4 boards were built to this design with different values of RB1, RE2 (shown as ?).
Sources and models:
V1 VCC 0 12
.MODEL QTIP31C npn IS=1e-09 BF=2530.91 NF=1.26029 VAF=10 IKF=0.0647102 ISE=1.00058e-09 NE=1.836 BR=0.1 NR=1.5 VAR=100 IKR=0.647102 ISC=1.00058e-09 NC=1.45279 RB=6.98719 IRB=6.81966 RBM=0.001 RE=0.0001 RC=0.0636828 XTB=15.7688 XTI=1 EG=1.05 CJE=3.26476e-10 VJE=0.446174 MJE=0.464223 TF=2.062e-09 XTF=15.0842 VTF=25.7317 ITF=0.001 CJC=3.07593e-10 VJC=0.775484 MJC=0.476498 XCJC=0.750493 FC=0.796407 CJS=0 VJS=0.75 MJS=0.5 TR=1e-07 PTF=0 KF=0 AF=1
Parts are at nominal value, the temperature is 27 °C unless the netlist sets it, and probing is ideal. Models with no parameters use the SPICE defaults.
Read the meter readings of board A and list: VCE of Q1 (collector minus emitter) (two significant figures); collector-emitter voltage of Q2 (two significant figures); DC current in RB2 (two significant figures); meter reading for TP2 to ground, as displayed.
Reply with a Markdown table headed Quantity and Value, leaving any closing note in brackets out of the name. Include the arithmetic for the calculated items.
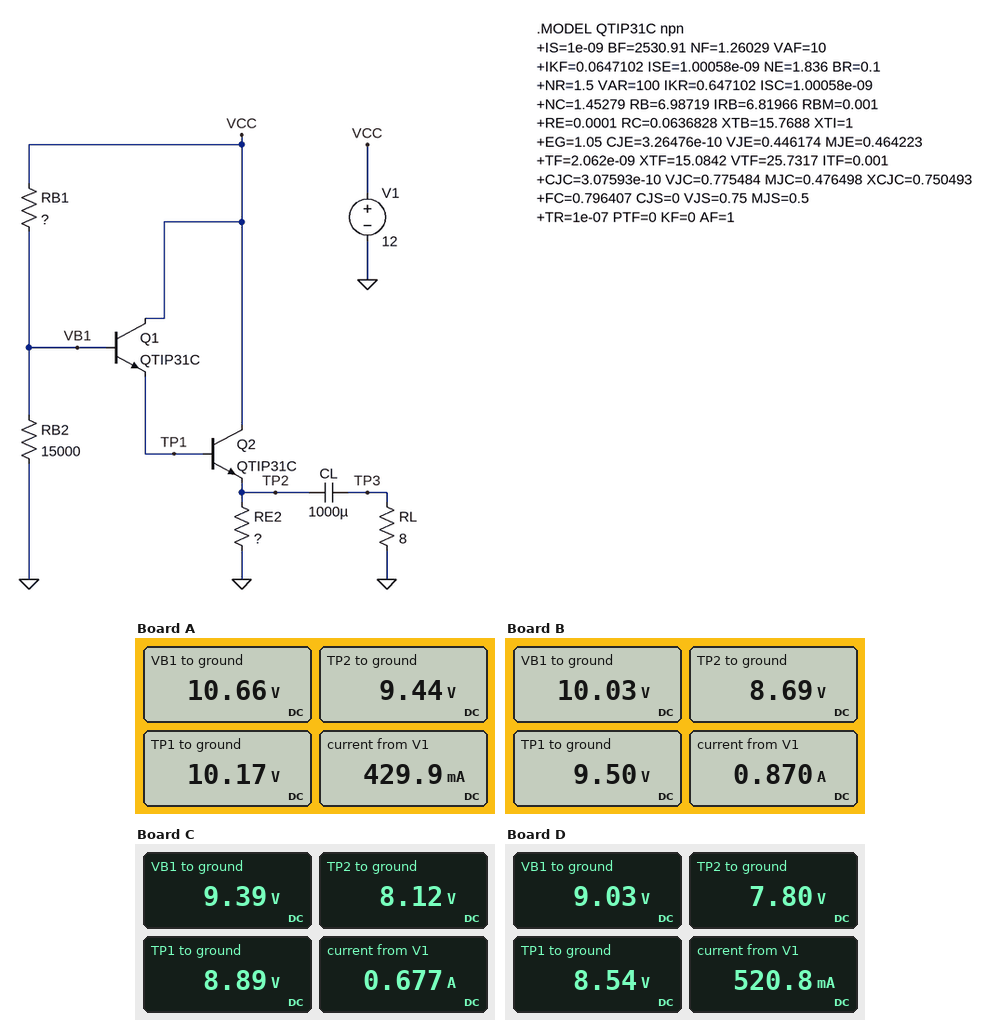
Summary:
| Quantity | Value |
|---|---|
| VCE of Q1 (collector minus emitter) | 12 V - 10.17 V = 1.8 V |
| collector-emitter voltage of Q2 | 12 V - 9.44 V = 2.6 V |
| DC current in RB2 | (10.66 V) / 15 kΩ = 710 µA |
| meter reading for TP2 to ground, as displayed | 9.44 V |
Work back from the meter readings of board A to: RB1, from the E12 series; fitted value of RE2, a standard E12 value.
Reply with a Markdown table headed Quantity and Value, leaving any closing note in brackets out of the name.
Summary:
| Quantity | Value |
|---|---|
| RB1, from the E12 series | 1.8 kΩ |
| fitted value of RE2, a standard E12 value | 22 Ω |
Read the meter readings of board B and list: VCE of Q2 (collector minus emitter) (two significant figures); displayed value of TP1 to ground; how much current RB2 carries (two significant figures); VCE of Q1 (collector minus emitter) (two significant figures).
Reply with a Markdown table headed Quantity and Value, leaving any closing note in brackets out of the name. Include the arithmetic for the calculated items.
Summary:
| Quantity | Value |
|---|---|
| VCE of Q2 (collector minus emitter) | 12 V - 8.69 V = 3.3 V |
| displayed value of TP1 to ground | 9.50 V |
| how much current RB2 carries | (10.03 V) / 15 kΩ = 670 µA |
| VCE of Q1 (collector minus emitter) | 12 V - 9.5 V = 2.5 V |
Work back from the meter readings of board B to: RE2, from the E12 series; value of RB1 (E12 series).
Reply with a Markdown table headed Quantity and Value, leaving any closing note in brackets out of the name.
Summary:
| Quantity | Value |
|---|---|
| RE2, from the E12 series | 10 Ω |
| value of RB1 | 2.7 kΩ |
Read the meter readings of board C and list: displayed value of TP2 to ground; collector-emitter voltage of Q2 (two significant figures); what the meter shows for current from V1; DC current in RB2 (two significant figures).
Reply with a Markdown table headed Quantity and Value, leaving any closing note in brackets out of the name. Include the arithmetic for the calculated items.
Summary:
| Quantity | Value |
|---|---|
| displayed value of TP2 to ground | 8.12 V |
| collector-emitter voltage of Q2 | 12 V - 8.12 V = 3.9 V |
| what the meter shows for current from V1 | 0.677 A |
| DC current in RB2 | (9.39 V) / 15 kΩ = 630 µA |
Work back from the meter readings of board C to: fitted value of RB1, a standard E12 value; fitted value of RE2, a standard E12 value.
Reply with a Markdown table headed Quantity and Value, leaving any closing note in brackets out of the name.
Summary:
| Quantity | Value |
|---|---|
| fitted value of RB1, a standard E12 value | 3.9 kΩ |
| fitted value of RE2, a standard E12 value | 12 Ω |
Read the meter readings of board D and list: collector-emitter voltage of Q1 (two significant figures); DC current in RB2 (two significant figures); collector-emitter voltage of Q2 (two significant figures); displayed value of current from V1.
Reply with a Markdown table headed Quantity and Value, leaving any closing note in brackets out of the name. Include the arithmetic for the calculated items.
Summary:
| Quantity | Value |
|---|---|
| collector-emitter voltage of Q1 | 12 V - 8.54 V = 3.5 V |
| DC current in RB2 | (9.03 V) / 15 kΩ = 600 µA |
| collector-emitter voltage of Q2 | 12 V - 7.8 V = 4.2 V |
| displayed value of current from V1 | 520.8 mA |
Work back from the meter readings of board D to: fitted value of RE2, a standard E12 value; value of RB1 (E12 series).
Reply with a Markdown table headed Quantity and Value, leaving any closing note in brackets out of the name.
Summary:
| Quantity | Value |
|---|---|
| fitted value of RE2, a standard E12 value | 15 Ω |
| value of RB1 | 4.7 kΩ |
